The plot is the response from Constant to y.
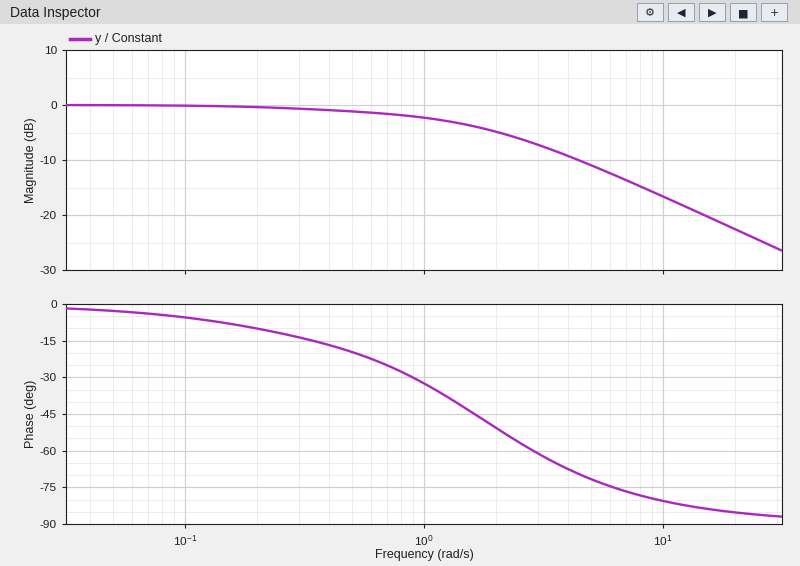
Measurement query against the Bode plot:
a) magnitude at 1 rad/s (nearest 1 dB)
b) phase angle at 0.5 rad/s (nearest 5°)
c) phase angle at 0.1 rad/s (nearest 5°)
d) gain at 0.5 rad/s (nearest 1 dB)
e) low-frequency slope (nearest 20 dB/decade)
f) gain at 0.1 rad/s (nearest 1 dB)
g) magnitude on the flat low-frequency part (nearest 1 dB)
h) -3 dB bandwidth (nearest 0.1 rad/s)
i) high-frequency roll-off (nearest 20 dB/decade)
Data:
-2 dB
-20°
-5°
-1 dB
0 dB/decade
0 dB
0 dB
1.3 rad/s
-20 dB/decade
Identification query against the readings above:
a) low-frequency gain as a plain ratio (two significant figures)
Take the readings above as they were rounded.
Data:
1.0
